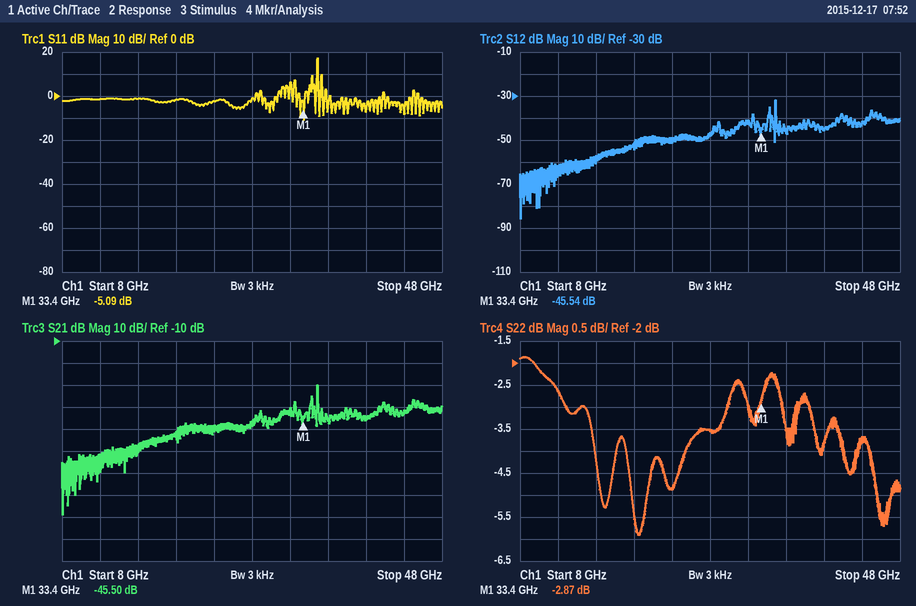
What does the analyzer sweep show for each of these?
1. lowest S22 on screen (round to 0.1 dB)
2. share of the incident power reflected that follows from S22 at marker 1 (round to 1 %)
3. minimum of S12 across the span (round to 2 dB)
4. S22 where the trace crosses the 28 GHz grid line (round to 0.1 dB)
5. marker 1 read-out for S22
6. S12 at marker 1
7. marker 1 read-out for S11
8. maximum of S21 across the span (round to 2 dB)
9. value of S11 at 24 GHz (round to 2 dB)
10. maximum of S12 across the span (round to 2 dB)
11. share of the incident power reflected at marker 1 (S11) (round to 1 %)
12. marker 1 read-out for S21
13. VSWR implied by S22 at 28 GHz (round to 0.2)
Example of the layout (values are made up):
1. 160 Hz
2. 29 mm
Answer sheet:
1. -5.9 dB
2. 52 %
3. -86 dB
4. -3.5 dB
5. -2.87 dB
6. -45.54 dB
7. -5.09 dB
8. -30 dB
9. -2 dB
10. -32 dB
11. 31 %
12. -45.50 dB
13. 5.0
